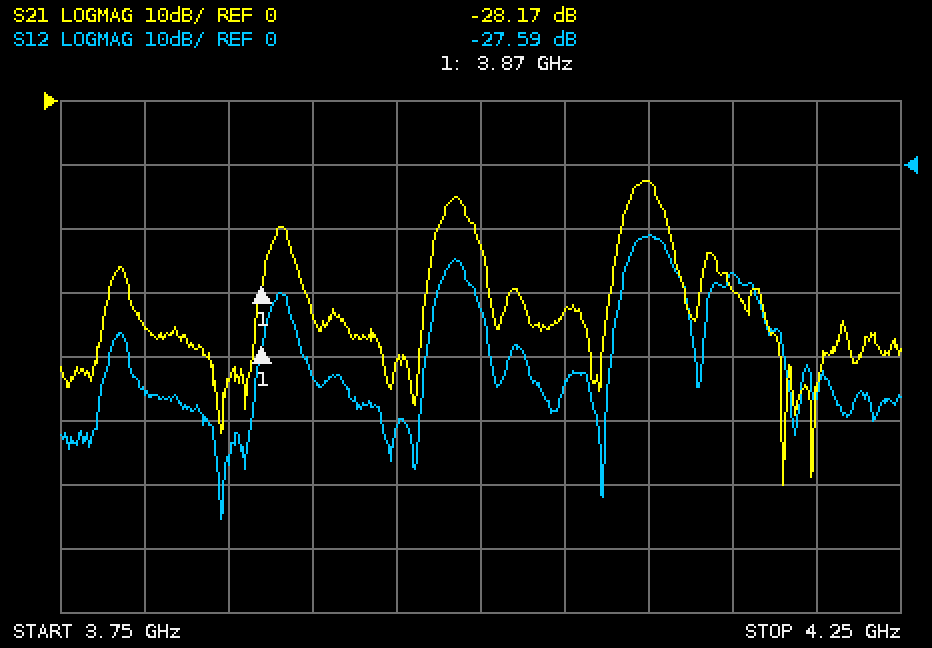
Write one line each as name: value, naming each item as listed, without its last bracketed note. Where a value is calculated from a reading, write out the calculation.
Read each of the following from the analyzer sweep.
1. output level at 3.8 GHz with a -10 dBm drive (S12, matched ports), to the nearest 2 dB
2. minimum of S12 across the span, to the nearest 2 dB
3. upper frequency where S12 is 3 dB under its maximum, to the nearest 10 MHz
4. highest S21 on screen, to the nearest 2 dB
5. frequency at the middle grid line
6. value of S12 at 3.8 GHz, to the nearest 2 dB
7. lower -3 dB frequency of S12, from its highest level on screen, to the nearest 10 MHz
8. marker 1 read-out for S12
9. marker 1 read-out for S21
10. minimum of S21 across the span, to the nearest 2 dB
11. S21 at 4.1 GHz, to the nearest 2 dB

output level at 3.8 GHz with a -10 dBm drive (S12, matched ports), to the nearest 2 dB: -10 dBm + (-36 dB) = -46 dBm
minimum of S12 across the span, to the nearest 2 dB: -56 dB
upper frequency where S12 is 3 dB under its maximum, to the nearest 10 MHz: 4.11 GHz
highest S21 on screen, to the nearest 2 dB: -12 dB
frequency at the middle grid line: 4 GHz
value of S12 at 3.8 GHz, to the nearest 2 dB: -36 dB
lower -3 dB frequency of S12, from its highest level on screen, to the nearest 10 MHz: 4.09 GHz
marker 1 read-out for S12: -27.59 dB
marker 1 read-out for S21: -28.17 dB
minimum of S21 across the span, to the nearest 2 dB: -60 dB
S21 at 4.1 GHz, to the nearest 2 dB: -12 dB
